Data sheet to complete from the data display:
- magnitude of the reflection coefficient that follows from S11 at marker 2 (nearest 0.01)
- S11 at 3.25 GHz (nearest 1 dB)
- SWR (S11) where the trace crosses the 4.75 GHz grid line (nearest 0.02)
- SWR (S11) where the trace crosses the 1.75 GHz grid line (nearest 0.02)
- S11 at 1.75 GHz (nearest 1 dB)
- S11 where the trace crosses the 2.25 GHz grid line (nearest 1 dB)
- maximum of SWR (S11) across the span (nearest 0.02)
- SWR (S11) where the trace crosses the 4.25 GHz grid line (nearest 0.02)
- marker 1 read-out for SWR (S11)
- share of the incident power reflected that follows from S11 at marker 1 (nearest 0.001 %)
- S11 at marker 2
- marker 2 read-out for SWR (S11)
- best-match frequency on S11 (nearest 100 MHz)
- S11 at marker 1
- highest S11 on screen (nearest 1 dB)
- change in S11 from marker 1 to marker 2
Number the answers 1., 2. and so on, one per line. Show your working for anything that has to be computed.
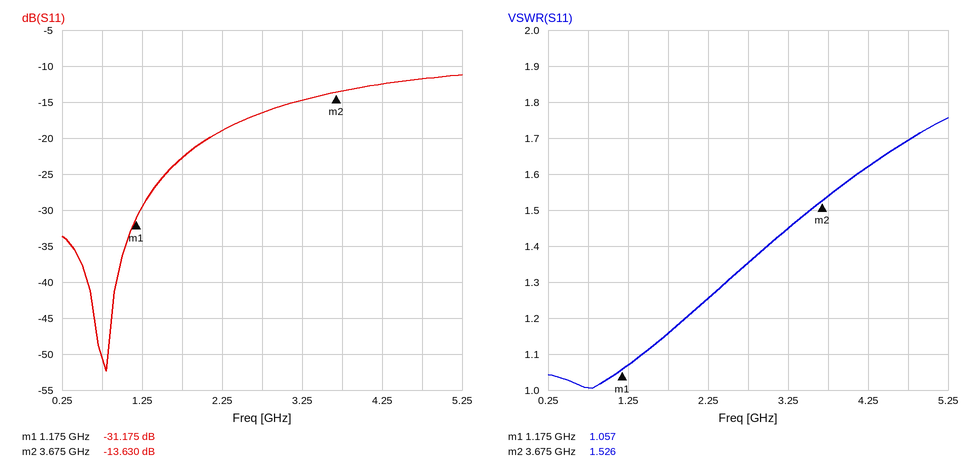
1. 10^(-13.63/20) ≈ 0.21
2. -15 dB
3. 1.70
4. 1.16
5. -23 dB
6. -19 dB
7. 1.76
8. 1.62
9. 1.057
10. 10^(-31.175/10) ≈ 0.076 %
11. -13.630 dB
12. 1.526
13. 800 MHz
14. -31.175 dB
15. -11 dB
16. -13.63 − (-31.175) = 17.545 dB
